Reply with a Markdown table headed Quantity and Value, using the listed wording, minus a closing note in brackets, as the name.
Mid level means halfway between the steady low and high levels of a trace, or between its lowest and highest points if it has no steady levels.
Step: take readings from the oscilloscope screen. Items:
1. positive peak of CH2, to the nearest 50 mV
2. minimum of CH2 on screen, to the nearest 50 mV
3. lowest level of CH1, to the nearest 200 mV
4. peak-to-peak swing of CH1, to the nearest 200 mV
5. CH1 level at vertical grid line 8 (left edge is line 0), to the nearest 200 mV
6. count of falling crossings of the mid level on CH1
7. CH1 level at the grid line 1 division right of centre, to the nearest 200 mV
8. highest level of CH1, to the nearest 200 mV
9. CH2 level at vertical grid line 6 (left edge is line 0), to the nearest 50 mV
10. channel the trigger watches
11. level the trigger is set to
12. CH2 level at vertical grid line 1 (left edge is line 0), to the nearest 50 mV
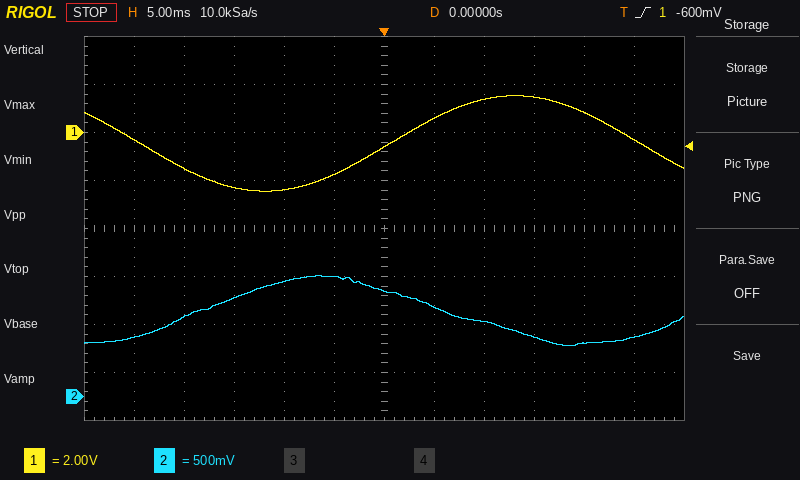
| Quantity | Value |
|---|---|
| positive peak of CH2, to the nearest 50 mV | 1.25 V |
| minimum of CH2 on screen, to the nearest 50 mV | 550 mV |
| lowest level of CH1, to the nearest 200 mV | -2.4 V |
| peak-to-peak swing of CH1, to the nearest 200 mV | 4.0 V |
| CH1 level at vertical grid line 8 (left edge is line 0), to the nearest 200 mV | 1.4 V |
| count of falling crossings of the mid level on CH1 | 2 |
| CH1 level at the grid line 1 division right of centre, to the nearest 200 mV | 600 mV |
| highest level of CH1, to the nearest 200 mV | 1.6 V |
| CH2 level at vertical grid line 6 (left edge is line 0), to the nearest 50 mV | 1.10 V |
| channel the trigger watches | CH1 |
| level the trigger is set to | -600 mV |
| CH2 level at vertical grid line 1 (left edge is line 0), to the nearest 50 mV | 600 mV |
